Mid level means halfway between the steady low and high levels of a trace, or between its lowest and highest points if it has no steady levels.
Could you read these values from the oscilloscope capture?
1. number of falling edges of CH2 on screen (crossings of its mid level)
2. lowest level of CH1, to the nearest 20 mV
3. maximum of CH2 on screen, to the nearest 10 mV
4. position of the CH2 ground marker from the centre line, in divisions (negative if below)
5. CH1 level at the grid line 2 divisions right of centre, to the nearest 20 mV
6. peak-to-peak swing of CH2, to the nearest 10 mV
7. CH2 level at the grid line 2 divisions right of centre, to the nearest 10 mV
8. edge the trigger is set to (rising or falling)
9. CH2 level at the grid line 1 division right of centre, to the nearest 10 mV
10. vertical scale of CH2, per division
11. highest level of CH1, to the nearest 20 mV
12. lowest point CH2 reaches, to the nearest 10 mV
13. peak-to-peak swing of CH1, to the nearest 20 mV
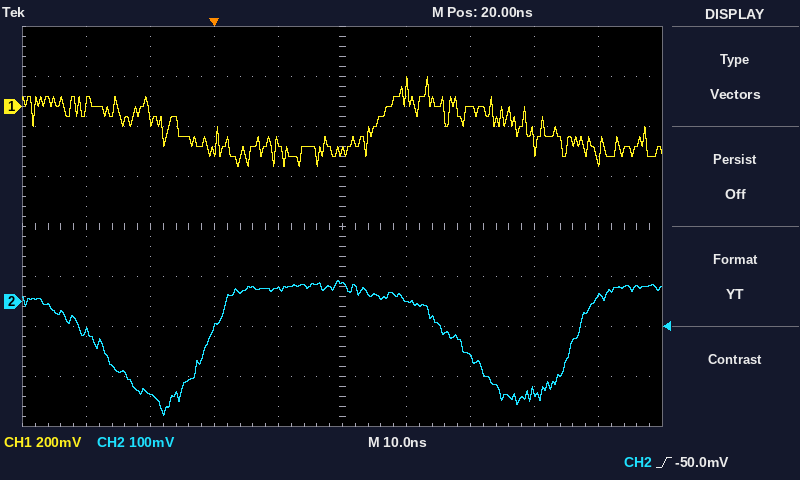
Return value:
2
-240 mV
40 mV
-1.5 div
0 mV
270 mV
-110 mV
rising
0 mV
100 mV
120 mV
-230 mV
360 mV
